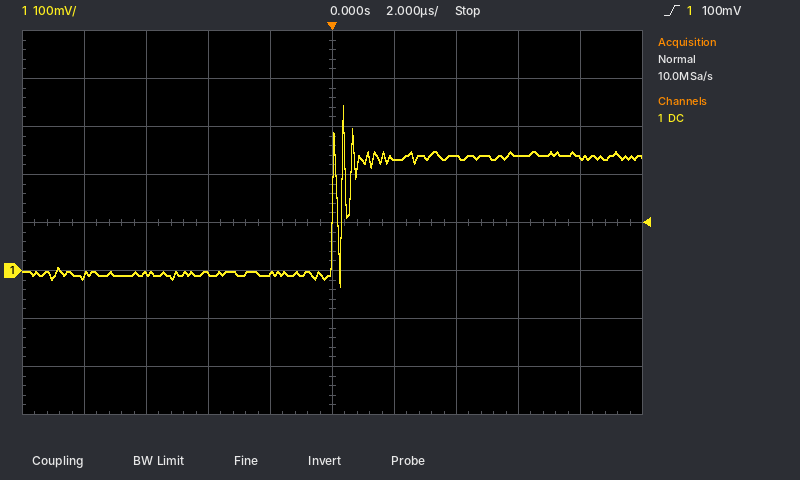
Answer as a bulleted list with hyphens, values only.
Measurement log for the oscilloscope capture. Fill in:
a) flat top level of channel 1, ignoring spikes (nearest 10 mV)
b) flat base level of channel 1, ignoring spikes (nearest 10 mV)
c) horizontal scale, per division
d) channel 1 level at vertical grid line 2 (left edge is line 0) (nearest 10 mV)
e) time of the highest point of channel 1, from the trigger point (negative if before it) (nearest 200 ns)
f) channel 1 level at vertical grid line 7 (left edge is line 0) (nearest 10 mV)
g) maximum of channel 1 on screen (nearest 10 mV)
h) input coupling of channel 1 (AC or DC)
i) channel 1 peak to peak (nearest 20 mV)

- 240 mV
- -10 mV
- 2 µs
- -10 mV
- +400 ns
- 240 mV
- 340 mV
- DC
- 380 mV
